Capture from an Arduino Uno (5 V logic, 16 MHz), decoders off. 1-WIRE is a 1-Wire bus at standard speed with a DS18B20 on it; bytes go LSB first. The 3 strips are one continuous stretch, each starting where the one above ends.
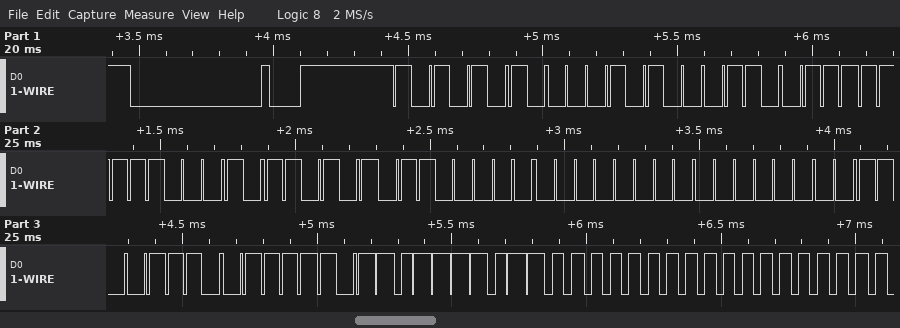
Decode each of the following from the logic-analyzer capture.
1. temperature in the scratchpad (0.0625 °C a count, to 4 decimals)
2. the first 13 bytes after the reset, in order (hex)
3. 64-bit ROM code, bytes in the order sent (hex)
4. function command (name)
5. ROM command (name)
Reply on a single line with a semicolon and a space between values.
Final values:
27.8125 °C; 55 28 E6 1F AD 06 00 00 73 BE BD 01 00; 28 E6 1F AD 06 00 00 73; Read Scratchpad; Match ROM
